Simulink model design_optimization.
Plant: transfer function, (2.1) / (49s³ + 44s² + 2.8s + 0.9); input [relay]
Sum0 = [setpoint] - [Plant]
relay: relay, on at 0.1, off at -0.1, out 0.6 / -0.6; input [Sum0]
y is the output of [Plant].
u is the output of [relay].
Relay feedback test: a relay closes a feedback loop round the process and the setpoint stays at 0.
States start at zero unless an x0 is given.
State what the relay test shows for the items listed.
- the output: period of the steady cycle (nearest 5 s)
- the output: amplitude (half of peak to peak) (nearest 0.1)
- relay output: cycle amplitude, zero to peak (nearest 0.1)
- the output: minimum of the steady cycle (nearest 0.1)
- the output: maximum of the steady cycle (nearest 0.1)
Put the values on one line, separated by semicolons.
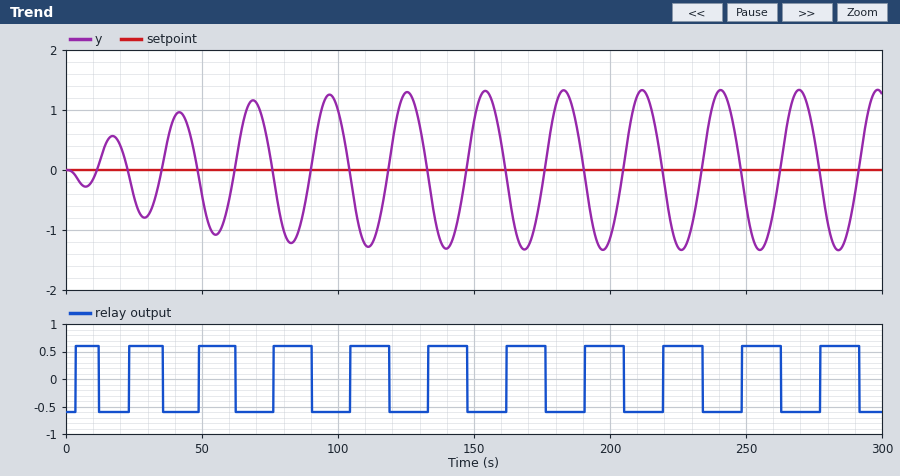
30 s; 1.3; 0.6; -1.3; 1.3
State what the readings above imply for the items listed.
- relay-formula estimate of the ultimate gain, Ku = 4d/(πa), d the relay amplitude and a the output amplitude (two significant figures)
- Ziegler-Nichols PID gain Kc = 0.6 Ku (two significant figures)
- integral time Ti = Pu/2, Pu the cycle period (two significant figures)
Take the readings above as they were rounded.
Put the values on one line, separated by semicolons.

0.59; 0.35; 15 s
